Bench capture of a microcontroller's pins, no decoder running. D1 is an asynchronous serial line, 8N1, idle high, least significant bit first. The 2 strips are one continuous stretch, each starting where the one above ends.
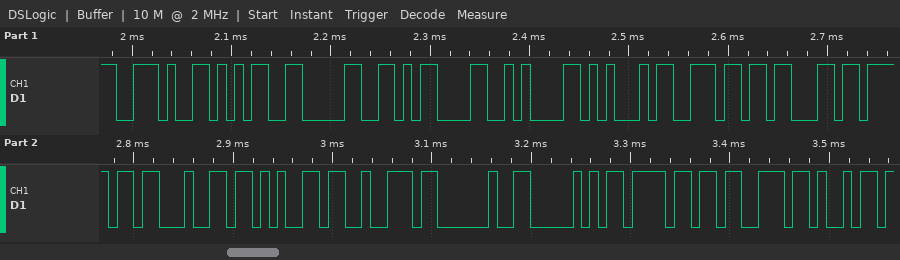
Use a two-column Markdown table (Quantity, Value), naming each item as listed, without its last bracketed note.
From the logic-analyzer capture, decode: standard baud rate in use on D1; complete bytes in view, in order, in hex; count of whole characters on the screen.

| Quantity | Value |
|---|---|
| standard baud rate in use on D1 | 115200 baud |
| complete bytes in view, in order, in hex | 0x2E 0x35 0x30 0x0D 0x0A 0x45 0x6E 0x63 0x6F 0x64 0x65 0x72 0x20 0x50 0x6F 0x73 0x69 |
| count of whole characters on the screen | 17 |
